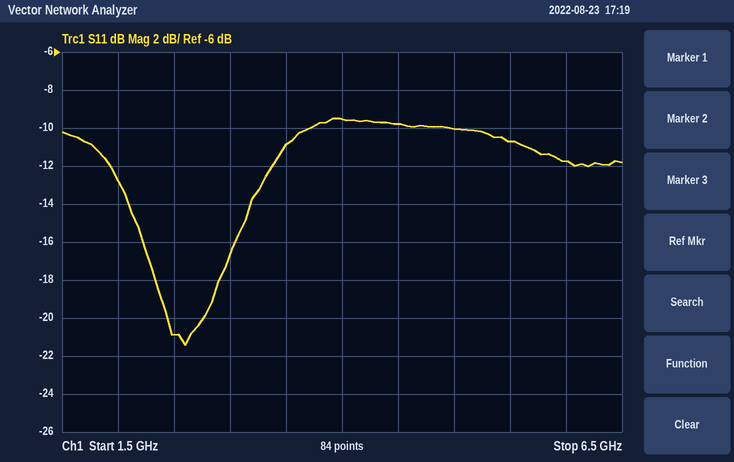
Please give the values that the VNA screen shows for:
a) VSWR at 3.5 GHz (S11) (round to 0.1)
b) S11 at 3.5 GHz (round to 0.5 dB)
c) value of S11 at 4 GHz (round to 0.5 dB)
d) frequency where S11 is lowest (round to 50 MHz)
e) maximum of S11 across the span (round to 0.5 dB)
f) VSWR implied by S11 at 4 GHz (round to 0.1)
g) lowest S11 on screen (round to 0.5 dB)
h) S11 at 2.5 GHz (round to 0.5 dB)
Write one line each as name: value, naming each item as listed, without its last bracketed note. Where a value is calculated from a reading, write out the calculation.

VSWR at 3.5 GHz (S11): |Γ| = 10^(-11/20) = 0.2818; VSWR = (1 + 0.2818)/(1 − 0.2818) ≈ 1.8
S11 at 3.5 GHz: -11.0 dB
value of S11 at 4 GHz: -9.5 dB
frequency where S11 is lowest: 2.60 GHz
maximum of S11 across the span: -9.5 dB
VSWR implied by S11 at 4 GHz: |Γ| = 10^(-9.5/20) = 0.3350; VSWR = (1 + 0.3350)/(1 − 0.3350) ≈ 2.0
lowest S11 on screen: -21.5 dB
S11 at 2.5 GHz: -21.0 dB
